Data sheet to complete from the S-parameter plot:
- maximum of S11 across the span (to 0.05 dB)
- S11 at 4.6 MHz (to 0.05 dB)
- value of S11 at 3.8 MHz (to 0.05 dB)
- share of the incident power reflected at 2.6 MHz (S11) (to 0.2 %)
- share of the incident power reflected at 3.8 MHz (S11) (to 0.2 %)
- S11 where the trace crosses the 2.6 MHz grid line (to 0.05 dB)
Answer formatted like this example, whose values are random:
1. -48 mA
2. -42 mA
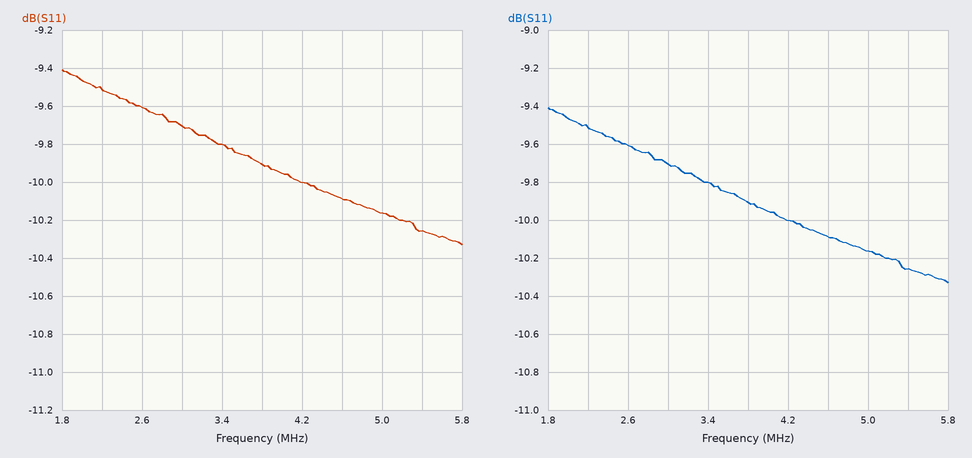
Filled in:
1. -9.40 dB
2. -10.10 dB
3. -9.90 dB
4. 11.0 %
5. 10.2 %
6. -9.60 dB
